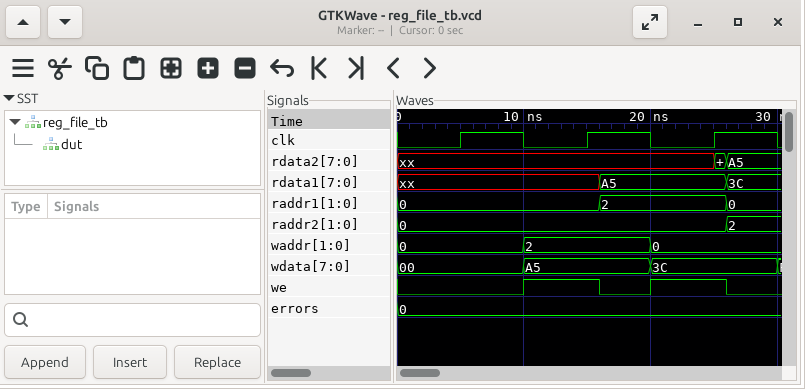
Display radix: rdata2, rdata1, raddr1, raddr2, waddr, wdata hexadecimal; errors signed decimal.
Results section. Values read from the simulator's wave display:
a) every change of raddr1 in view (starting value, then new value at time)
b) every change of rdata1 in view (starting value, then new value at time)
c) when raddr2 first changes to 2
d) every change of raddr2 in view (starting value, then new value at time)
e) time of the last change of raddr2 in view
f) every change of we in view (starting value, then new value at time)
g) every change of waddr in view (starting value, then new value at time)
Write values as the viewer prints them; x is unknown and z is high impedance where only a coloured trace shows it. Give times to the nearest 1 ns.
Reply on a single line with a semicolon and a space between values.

0, 2 at 16 ns, 0 at 26 ns; xx, A5 at 16 ns, 3C at 26 ns; 26 ns; 0, 2 at 26 ns; 26 ns; 0, 1 at 10 ns, 0 at 16 ns, 1 at 20 ns, 0 at 26 ns; 0, 2 at 10 ns, 0 at 20 ns
